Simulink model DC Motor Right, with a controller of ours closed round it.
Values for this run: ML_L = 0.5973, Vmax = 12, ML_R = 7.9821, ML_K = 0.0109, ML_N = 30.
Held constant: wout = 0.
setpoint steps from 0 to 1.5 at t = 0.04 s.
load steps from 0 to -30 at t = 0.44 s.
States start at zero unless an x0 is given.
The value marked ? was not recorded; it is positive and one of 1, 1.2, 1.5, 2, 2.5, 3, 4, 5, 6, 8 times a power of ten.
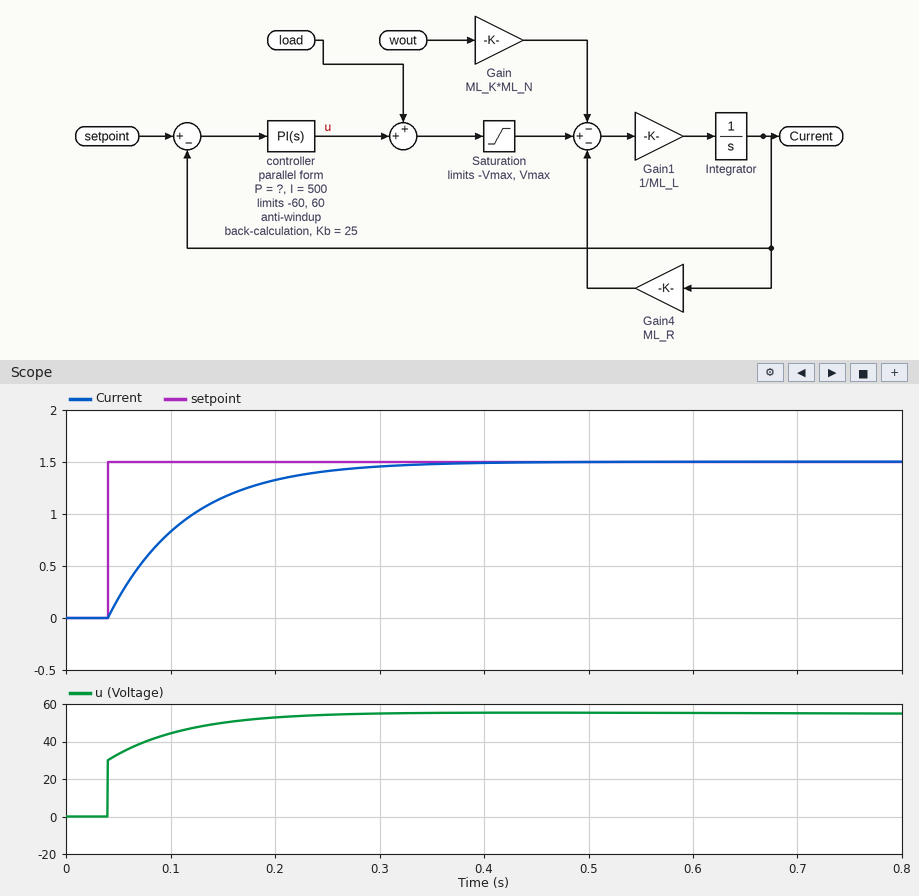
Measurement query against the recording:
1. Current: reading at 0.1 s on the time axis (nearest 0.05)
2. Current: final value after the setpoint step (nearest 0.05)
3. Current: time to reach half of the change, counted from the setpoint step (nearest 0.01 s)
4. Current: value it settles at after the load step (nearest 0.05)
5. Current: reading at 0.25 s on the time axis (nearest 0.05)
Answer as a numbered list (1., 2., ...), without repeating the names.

1. 0.85
2. 1.50
3. 0.05 s
4. 1.50
5. 1.40
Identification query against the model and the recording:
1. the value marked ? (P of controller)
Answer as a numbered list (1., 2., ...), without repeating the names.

1. 20
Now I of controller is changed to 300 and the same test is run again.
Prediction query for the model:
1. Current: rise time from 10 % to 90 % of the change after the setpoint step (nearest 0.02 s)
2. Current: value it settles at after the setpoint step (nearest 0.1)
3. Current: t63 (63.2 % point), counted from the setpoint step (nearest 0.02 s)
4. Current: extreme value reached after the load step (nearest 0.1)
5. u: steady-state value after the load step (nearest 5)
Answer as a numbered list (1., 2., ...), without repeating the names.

1. 0.16 s
2. 1.5
3. 0.08 s
4. 1.3
5. 40
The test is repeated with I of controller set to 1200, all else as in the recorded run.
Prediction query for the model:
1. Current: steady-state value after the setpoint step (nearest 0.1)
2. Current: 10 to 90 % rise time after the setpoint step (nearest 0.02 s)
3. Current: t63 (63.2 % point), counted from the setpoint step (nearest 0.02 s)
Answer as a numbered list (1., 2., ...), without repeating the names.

1. 1.5
2. 0.16 s
3. 0.08 s
